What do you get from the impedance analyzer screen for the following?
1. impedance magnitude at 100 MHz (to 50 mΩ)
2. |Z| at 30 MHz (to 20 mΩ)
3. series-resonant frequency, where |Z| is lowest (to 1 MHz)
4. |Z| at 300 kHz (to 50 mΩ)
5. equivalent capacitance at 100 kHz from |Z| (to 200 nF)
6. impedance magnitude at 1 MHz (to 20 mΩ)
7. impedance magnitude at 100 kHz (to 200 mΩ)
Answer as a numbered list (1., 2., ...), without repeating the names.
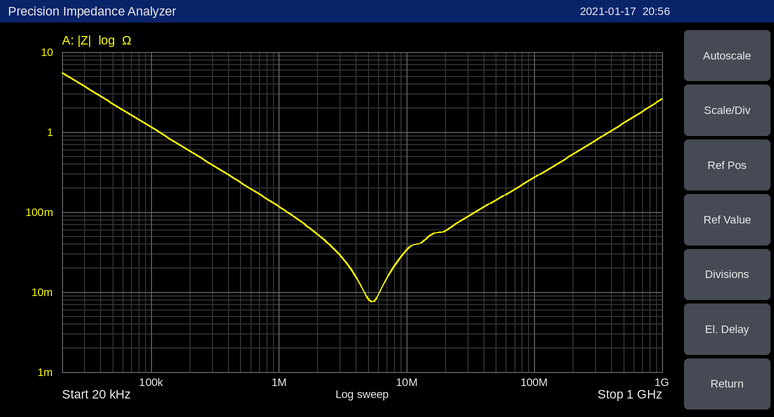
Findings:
1. 250 mΩ
2. 80 mΩ
3. 5 MHz
4. 400 mΩ
5. 1.4 µF
6. 120 mΩ
7. 1.2 Ω
